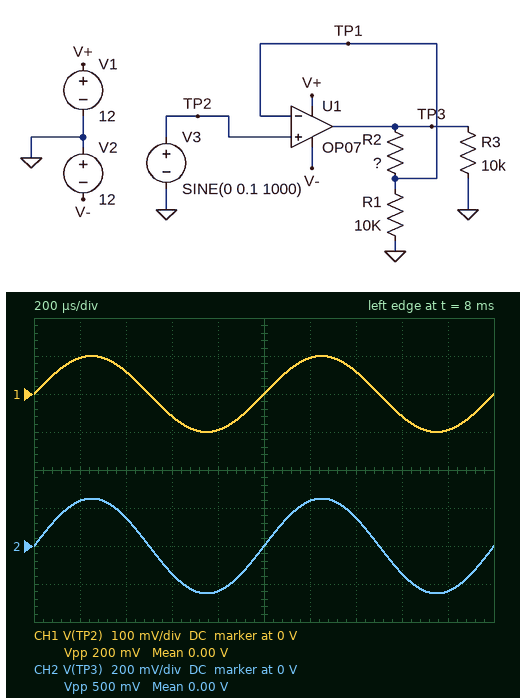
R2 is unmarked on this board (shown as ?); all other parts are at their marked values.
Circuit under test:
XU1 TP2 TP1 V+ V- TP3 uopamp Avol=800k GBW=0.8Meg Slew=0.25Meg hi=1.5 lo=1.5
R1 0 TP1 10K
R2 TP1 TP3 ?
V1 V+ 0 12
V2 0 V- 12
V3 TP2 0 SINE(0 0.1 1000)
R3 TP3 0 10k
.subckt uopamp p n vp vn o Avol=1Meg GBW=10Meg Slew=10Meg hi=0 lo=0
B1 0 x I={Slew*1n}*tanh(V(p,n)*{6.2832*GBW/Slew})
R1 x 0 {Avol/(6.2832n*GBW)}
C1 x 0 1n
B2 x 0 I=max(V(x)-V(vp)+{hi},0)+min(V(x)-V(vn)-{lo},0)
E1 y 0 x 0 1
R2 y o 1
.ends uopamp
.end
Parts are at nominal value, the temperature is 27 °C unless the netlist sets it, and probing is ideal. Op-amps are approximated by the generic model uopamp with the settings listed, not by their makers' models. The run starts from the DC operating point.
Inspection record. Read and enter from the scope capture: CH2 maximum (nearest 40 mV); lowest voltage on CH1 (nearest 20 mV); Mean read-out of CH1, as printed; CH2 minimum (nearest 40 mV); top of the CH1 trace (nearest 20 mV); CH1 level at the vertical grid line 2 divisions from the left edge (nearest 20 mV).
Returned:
240 mV
-100 mV
0.00 V
-240 mV
100 mV
60 mV
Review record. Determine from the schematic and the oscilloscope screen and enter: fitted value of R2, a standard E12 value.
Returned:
15 kΩ
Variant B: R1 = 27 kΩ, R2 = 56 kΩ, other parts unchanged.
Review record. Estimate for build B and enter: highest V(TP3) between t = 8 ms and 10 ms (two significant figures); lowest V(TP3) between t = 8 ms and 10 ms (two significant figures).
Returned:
310 mV
-310 mV
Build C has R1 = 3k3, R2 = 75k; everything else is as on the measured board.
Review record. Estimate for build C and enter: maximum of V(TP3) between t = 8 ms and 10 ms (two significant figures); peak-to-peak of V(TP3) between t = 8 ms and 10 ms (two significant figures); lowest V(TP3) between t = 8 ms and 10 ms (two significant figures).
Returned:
2.4 V
4.7 V
-2.4 V
